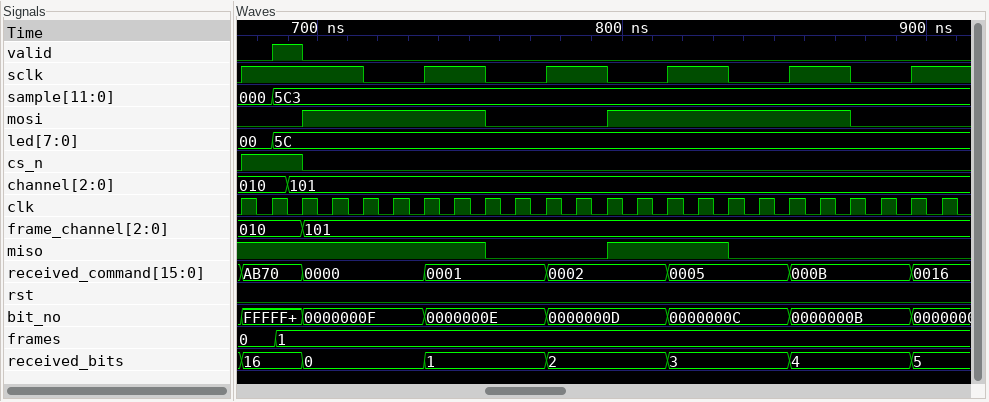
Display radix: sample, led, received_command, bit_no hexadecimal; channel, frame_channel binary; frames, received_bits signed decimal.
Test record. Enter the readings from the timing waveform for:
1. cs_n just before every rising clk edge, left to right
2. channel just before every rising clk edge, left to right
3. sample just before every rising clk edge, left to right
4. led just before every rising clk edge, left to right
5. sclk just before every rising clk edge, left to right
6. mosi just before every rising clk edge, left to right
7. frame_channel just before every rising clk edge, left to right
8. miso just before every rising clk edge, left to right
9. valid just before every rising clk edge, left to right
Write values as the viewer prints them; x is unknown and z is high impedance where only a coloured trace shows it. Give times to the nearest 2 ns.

0 1 1 0 0 0 0 0 0 0 0 0 0 0 0 0 0 0 0 0 0 0 0 0
010, 010, 101, 101, 101, 101, 101, 101, 101, 101, 101, 101, 101, 101, 101, 101, 101, 101, 101, 101, 101, 101, 101, 101
000, 000, 5C3, 5C3, 5C3, 5C3, 5C3, 5C3, 5C3, 5C3, 5C3, 5C3, 5C3, 5C3, 5C3, 5C3, 5C3, 5C3, 5C3, 5C3, 5C3, 5C3, 5C3, 5C3
00, 00, 5C, 5C, 5C, 5C, 5C, 5C, 5C, 5C, 5C, 5C, 5C, 5C, 5C, 5C, 5C, 5C, 5C, 5C, 5C, 5C, 5C, 5C
0 1 1 1 1 0 0 1 1 0 0 1 1 0 0 1 1 0 0 1 1 0 0 1
0 0 0 1 1 1 1 1 1 0 0 0 0 1 1 1 1 1 1 1 1 0 0 0
010, 010, 010, 101, 101, 101, 101, 101, 101, 101, 101, 101, 101, 101, 101, 101, 101, 101, 101, 101, 101, 101, 101, 101
1 1 1 1 1 1 1 1 1 0 0 0 0 1 1 1 1 0 0 0 0 0 0 0
0 0 1 0 0 0 0 0 0 0 0 0 0 0 0 0 0 0 0 0 0 0 0 0
